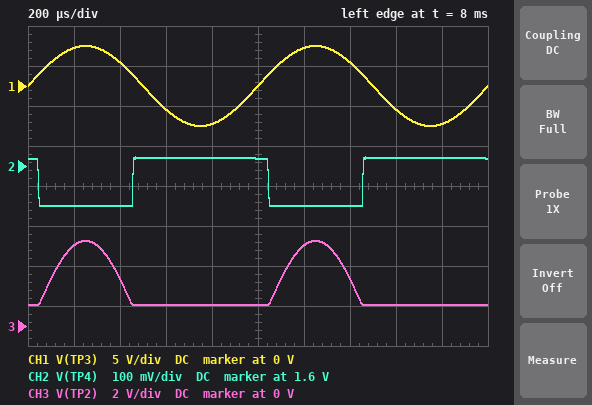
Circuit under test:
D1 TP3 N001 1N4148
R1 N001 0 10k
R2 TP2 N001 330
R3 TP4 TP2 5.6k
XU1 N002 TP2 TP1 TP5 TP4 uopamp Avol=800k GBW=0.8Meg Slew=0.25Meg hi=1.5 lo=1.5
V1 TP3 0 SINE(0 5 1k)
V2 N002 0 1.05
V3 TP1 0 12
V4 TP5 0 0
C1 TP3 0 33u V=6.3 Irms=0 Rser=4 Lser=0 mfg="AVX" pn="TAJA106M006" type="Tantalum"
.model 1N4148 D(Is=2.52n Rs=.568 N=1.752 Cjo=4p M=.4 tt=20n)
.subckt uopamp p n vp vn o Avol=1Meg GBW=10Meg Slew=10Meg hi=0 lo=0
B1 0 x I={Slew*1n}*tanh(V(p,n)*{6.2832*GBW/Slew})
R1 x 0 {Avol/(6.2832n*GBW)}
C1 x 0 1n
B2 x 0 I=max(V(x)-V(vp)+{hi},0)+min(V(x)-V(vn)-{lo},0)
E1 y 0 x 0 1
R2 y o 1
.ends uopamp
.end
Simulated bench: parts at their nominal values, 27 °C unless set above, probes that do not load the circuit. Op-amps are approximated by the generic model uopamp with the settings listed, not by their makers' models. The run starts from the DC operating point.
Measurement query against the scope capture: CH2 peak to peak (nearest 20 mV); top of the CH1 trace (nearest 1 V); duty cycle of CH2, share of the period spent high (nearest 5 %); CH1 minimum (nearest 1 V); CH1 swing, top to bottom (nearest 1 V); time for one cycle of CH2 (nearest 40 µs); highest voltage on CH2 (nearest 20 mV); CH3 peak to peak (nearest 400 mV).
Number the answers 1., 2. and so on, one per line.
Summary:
1. 120 mV
2. 5 V
3. 60 %
4. -5 V
5. 10 V
6. 1.00 ms
7. 1.62 V
8. 3.2 V
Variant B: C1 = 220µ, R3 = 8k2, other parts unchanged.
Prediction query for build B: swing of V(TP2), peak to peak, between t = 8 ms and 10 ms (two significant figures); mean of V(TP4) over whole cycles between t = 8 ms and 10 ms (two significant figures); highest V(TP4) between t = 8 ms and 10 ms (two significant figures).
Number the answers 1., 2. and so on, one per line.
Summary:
1. 3.3 V
2. 1.7 V
3. 1.9 V
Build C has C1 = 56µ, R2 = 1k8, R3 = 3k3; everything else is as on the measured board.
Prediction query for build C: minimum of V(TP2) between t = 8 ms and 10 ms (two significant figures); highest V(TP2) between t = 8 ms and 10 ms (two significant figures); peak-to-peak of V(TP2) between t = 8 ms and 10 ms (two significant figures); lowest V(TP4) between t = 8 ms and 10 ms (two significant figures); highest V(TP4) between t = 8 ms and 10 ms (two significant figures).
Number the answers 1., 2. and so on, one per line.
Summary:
1. 1.2 V
2. 3.4 V
3. 2.2 V
4. 1.5 V
5. 1.5 V
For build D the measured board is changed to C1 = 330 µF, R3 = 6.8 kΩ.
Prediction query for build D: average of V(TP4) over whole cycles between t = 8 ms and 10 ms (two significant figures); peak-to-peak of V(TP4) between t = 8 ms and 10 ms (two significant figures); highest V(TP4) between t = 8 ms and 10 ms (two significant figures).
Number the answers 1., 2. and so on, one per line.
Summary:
1. 1.6 V
2. 240 mV
3. 1.7 V
